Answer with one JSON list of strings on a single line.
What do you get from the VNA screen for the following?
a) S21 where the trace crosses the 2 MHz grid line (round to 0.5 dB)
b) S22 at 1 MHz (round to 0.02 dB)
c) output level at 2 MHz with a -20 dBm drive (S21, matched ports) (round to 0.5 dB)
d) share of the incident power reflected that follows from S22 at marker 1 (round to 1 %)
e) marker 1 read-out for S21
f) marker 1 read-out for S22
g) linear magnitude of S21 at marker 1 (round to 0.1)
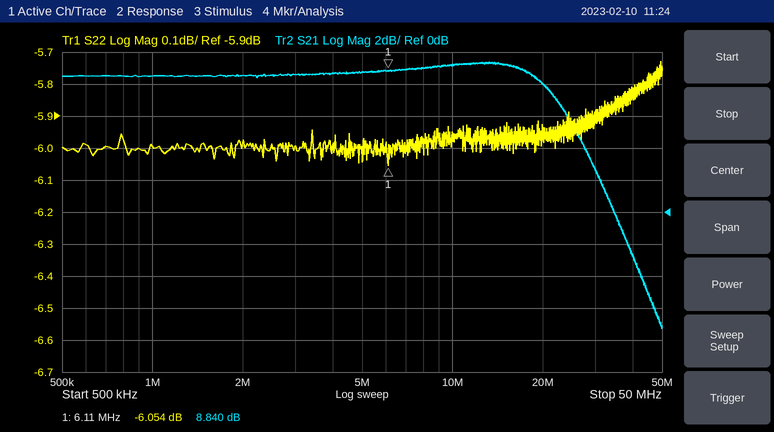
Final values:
["8.5 dB", "-6.00 dB", "-11.5 dBm", "25 %", "8.840 dB", "-6.054 dB", "2.8"]
